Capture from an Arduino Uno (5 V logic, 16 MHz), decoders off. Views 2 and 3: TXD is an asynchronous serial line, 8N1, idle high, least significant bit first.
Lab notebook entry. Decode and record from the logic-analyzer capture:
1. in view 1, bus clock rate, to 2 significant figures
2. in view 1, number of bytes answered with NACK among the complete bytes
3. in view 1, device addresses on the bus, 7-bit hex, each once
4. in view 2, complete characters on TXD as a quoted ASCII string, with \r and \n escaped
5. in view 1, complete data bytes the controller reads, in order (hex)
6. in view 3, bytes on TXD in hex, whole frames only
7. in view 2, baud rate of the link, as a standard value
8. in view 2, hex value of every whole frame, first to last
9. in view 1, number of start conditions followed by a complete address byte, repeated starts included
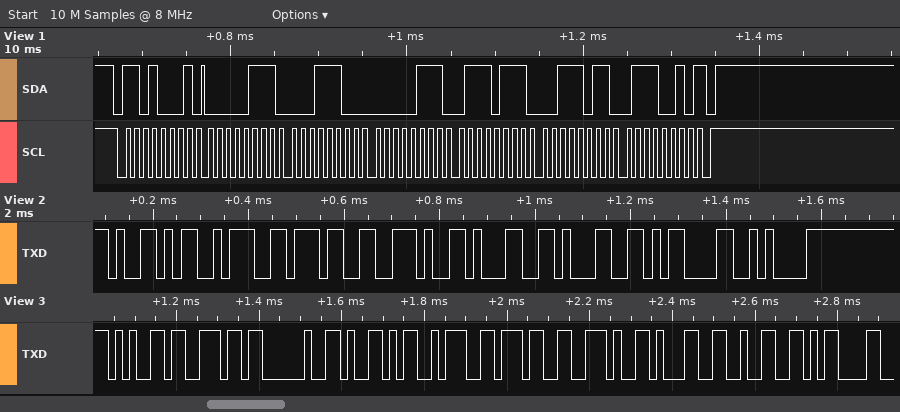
100 kHz
1
0x68
"Y:7.11\r\n"
07 1C 07 77 3B 72
65 6E 20 59 3A 37 2E 31 32 0D
57600 baud
59 3A 37 2E 31 31 0D 0A
1
